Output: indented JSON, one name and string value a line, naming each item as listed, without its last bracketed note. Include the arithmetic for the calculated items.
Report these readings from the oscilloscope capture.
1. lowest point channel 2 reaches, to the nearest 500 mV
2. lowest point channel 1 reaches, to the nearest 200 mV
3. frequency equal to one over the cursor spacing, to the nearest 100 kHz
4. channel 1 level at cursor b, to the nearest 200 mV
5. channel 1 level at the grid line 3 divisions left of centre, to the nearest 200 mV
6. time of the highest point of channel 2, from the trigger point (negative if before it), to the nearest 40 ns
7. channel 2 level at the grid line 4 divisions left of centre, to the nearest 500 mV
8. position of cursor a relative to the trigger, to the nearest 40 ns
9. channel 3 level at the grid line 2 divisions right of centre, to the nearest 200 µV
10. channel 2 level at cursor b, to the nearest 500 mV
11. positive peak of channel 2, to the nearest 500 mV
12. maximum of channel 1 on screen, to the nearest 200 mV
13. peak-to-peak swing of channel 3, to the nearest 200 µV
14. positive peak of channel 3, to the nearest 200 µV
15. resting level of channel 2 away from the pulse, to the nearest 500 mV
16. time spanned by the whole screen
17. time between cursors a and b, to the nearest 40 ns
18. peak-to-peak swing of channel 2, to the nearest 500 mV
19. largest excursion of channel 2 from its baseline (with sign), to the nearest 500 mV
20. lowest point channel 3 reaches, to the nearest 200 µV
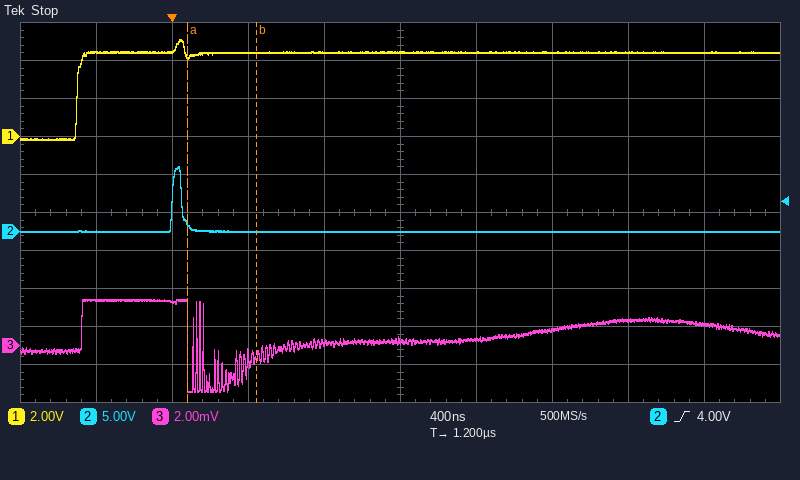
{
  "lowest point channel 2 reaches, to the nearest 500 mV": "0.0 V",
  "lowest point channel 1 reaches, to the nearest 200 mV": "-200 mV",
  "frequency equal to one over the cursor spacing, to the nearest 100 kHz": "1 / 360 ns ≈ 2.8 MHz",
  "channel 1 level at cursor b, to the nearest 200 mV": "4.4 V",
  "channel 1 level at the grid line 3 divisions left of centre, to the nearest 200 mV": "4.6 V",
  "time of the highest point of channel 2, from the trigger point (negative if before it), to the nearest 40 ns": "+40 ns",
  "channel 2 level at the grid line 4 divisions left of centre, to the nearest 500 mV": "0.0 V",
  "position of cursor a relative to the trigger, to the nearest 40 ns": "+80 ns",
  "channel 3 level at the grid line 2 divisions right of centre, to the nearest 200 µV": "800 µV",
  "channel 2 level at cursor b, to the nearest 500 mV": "0.0 V",
  "positive peak of channel 2, to the nearest 500 mV": "8.5 V",
  "maximum of channel 1 on screen, to the nearest 200 mV": "5.2 V",
  "peak-to-peak swing of channel 3, to the nearest 200 µV": "2.4 mV − (-2.4 mV) = 4.8 mV",
  "positive peak of channel 3, to the nearest 200 µV": "2.4 mV",
  "resting level of channel 2 away from the pulse, to the nearest 500 mV": "0.0 V",
  "time spanned by the whole screen": "4 µs",
  "time between cursors a and b, to the nearest 40 ns": "360 ns",
  "peak-to-peak swing of channel 2, to the nearest 500 mV": "8.5 V − (0.0 V) = 8.5 V",
  "largest excursion of channel 2 from its baseline (with sign), to the nearest 500 mV": "8.5 V − (0.0 V) = +8.5 V",
  "lowest point channel 3 reaches, to the nearest 200 µV": "-2.4 mV"
}
